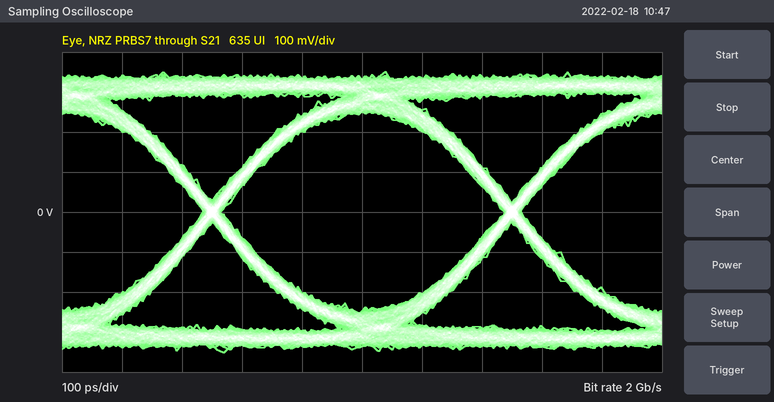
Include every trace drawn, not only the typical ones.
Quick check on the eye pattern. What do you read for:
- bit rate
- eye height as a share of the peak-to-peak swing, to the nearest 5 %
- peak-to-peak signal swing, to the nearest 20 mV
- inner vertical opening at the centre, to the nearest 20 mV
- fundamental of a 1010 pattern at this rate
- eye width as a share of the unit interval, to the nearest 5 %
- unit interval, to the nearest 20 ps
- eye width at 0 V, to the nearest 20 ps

2 Gb/s
70 %
700 mV
500 mV
1 GHz
95 %
500 ps
480 ps
